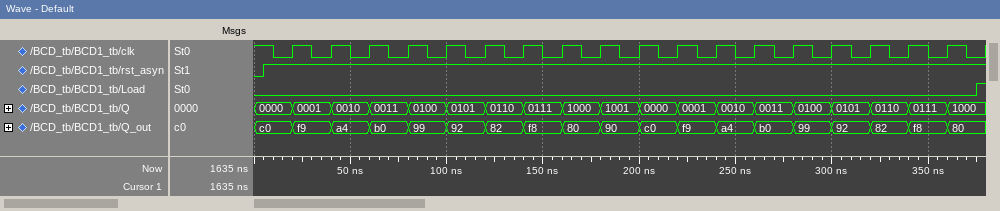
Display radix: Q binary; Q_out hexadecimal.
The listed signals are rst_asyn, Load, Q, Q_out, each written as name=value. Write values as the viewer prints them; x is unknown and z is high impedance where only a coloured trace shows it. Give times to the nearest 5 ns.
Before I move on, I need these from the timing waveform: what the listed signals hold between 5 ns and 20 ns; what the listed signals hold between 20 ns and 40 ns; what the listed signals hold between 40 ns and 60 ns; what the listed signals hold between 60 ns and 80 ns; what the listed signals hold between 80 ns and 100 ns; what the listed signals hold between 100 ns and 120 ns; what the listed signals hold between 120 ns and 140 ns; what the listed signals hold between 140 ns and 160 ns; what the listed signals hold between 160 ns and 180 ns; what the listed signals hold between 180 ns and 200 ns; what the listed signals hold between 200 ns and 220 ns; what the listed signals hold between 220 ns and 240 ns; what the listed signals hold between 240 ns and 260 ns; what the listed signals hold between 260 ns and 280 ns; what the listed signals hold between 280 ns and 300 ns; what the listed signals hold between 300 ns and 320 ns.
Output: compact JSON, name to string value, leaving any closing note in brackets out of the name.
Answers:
{"what the listed signals hold between 5 ns and 20 ns": "rst_asyn=1, Load=0, Q=0000, Q_out=c0", "what the listed signals hold between 20 ns and 40 ns": "rst_asyn=1, Load=0, Q=0001, Q_out=f9", "what the listed signals hold between 40 ns and 60 ns": "rst_asyn=1, Load=0, Q=0010, Q_out=a4", "what the listed signals hold between 60 ns and 80 ns": "rst_asyn=1, Load=0, Q=0011, Q_out=b0", "what the listed signals hold between 80 ns and 100 ns": "rst_asyn=1, Load=0, Q=0100, Q_out=99", "what the listed signals hold between 100 ns and 120 ns": "rst_asyn=1, Load=0, Q=0101, Q_out=92", "what the listed signals hold between 120 ns and 140 ns": "rst_asyn=1, Load=0, Q=0110, Q_out=82", "what the listed signals hold between 140 ns and 160 ns": "rst_asyn=1, Load=0, Q=0111, Q_out=f8", "what the listed signals hold between 160 ns and 180 ns": "rst_asyn=1, Load=0, Q=1000, Q_out=80", "what the listed signals hold between 180 ns and 200 ns": "rst_asyn=1, Load=0, Q=1001, Q_out=90", "what the listed signals hold between 200 ns and 220 ns": "rst_asyn=1, Load=0, Q=0000, Q_out=c0", "what the listed signals hold between 220 ns and 240 ns": "rst_asyn=1, Load=0, Q=0001, Q_out=f9", "what the listed signals hold between 240 ns and 260 ns": "rst_asyn=1, Load=0, Q=0010, Q_out=a4", "what the listed signals hold between 260 ns and 280 ns": "rst_asyn=1, Load=0, Q=0011, Q_out=b0", "what the listed signals hold between 280 ns and 300 ns": "rst_asyn=1, Load=0, Q=0100, Q_out=99", "what the listed signals hold between 300 ns and 320 ns": "rst_asyn=1, Load=0, Q=0101, Q_out=92"}
